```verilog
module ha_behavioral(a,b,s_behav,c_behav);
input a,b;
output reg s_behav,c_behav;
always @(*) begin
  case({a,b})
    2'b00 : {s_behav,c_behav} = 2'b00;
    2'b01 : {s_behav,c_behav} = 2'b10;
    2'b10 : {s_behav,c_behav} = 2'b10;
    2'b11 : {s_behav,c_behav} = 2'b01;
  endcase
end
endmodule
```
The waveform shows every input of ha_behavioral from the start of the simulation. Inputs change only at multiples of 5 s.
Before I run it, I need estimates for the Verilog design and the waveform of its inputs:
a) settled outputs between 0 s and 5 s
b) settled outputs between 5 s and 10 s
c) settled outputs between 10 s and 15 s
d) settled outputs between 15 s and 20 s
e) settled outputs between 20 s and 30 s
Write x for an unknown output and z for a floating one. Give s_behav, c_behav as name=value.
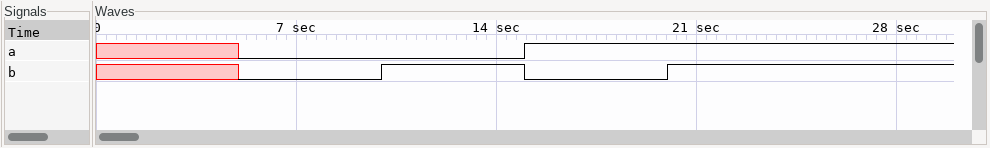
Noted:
s_behav=x, c_behav=x
s_behav=0, c_behav=0
s_behav=1, c_behav=0
s_behav=1, c_behav=0
s_behav=0, c_behav=1
